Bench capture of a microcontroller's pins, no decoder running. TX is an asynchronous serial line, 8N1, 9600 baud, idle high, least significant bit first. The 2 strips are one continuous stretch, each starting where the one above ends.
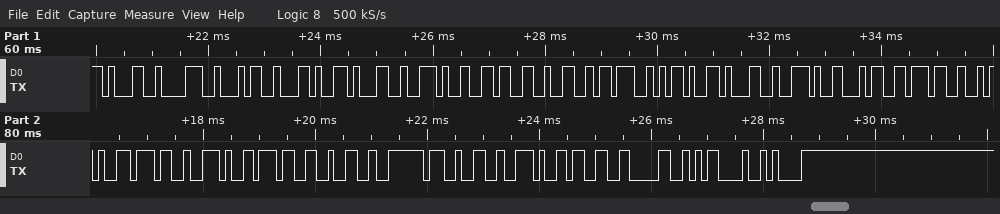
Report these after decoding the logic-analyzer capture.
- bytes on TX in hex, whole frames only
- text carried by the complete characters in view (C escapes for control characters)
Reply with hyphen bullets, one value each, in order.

- 31 38 34 2C 31 2E 36 32 3B 2D 31 2E 34 37 2A 37 2E 37 32 7E 32 2E 33 30 0D 0A
- "184,1.62;-1.47*7.72~2.30\r\n"
